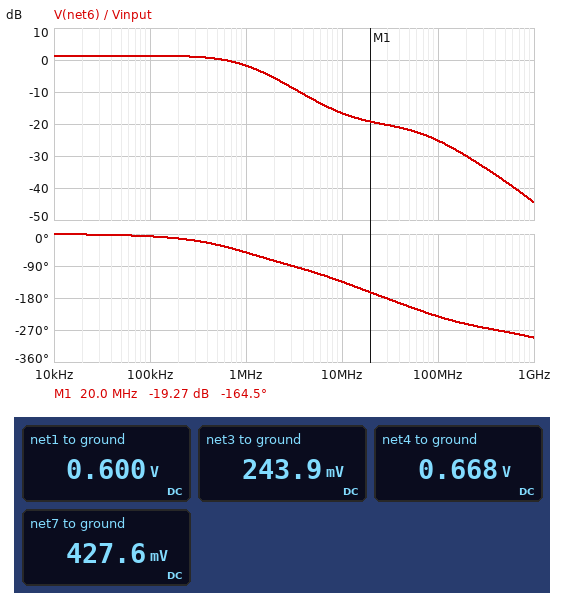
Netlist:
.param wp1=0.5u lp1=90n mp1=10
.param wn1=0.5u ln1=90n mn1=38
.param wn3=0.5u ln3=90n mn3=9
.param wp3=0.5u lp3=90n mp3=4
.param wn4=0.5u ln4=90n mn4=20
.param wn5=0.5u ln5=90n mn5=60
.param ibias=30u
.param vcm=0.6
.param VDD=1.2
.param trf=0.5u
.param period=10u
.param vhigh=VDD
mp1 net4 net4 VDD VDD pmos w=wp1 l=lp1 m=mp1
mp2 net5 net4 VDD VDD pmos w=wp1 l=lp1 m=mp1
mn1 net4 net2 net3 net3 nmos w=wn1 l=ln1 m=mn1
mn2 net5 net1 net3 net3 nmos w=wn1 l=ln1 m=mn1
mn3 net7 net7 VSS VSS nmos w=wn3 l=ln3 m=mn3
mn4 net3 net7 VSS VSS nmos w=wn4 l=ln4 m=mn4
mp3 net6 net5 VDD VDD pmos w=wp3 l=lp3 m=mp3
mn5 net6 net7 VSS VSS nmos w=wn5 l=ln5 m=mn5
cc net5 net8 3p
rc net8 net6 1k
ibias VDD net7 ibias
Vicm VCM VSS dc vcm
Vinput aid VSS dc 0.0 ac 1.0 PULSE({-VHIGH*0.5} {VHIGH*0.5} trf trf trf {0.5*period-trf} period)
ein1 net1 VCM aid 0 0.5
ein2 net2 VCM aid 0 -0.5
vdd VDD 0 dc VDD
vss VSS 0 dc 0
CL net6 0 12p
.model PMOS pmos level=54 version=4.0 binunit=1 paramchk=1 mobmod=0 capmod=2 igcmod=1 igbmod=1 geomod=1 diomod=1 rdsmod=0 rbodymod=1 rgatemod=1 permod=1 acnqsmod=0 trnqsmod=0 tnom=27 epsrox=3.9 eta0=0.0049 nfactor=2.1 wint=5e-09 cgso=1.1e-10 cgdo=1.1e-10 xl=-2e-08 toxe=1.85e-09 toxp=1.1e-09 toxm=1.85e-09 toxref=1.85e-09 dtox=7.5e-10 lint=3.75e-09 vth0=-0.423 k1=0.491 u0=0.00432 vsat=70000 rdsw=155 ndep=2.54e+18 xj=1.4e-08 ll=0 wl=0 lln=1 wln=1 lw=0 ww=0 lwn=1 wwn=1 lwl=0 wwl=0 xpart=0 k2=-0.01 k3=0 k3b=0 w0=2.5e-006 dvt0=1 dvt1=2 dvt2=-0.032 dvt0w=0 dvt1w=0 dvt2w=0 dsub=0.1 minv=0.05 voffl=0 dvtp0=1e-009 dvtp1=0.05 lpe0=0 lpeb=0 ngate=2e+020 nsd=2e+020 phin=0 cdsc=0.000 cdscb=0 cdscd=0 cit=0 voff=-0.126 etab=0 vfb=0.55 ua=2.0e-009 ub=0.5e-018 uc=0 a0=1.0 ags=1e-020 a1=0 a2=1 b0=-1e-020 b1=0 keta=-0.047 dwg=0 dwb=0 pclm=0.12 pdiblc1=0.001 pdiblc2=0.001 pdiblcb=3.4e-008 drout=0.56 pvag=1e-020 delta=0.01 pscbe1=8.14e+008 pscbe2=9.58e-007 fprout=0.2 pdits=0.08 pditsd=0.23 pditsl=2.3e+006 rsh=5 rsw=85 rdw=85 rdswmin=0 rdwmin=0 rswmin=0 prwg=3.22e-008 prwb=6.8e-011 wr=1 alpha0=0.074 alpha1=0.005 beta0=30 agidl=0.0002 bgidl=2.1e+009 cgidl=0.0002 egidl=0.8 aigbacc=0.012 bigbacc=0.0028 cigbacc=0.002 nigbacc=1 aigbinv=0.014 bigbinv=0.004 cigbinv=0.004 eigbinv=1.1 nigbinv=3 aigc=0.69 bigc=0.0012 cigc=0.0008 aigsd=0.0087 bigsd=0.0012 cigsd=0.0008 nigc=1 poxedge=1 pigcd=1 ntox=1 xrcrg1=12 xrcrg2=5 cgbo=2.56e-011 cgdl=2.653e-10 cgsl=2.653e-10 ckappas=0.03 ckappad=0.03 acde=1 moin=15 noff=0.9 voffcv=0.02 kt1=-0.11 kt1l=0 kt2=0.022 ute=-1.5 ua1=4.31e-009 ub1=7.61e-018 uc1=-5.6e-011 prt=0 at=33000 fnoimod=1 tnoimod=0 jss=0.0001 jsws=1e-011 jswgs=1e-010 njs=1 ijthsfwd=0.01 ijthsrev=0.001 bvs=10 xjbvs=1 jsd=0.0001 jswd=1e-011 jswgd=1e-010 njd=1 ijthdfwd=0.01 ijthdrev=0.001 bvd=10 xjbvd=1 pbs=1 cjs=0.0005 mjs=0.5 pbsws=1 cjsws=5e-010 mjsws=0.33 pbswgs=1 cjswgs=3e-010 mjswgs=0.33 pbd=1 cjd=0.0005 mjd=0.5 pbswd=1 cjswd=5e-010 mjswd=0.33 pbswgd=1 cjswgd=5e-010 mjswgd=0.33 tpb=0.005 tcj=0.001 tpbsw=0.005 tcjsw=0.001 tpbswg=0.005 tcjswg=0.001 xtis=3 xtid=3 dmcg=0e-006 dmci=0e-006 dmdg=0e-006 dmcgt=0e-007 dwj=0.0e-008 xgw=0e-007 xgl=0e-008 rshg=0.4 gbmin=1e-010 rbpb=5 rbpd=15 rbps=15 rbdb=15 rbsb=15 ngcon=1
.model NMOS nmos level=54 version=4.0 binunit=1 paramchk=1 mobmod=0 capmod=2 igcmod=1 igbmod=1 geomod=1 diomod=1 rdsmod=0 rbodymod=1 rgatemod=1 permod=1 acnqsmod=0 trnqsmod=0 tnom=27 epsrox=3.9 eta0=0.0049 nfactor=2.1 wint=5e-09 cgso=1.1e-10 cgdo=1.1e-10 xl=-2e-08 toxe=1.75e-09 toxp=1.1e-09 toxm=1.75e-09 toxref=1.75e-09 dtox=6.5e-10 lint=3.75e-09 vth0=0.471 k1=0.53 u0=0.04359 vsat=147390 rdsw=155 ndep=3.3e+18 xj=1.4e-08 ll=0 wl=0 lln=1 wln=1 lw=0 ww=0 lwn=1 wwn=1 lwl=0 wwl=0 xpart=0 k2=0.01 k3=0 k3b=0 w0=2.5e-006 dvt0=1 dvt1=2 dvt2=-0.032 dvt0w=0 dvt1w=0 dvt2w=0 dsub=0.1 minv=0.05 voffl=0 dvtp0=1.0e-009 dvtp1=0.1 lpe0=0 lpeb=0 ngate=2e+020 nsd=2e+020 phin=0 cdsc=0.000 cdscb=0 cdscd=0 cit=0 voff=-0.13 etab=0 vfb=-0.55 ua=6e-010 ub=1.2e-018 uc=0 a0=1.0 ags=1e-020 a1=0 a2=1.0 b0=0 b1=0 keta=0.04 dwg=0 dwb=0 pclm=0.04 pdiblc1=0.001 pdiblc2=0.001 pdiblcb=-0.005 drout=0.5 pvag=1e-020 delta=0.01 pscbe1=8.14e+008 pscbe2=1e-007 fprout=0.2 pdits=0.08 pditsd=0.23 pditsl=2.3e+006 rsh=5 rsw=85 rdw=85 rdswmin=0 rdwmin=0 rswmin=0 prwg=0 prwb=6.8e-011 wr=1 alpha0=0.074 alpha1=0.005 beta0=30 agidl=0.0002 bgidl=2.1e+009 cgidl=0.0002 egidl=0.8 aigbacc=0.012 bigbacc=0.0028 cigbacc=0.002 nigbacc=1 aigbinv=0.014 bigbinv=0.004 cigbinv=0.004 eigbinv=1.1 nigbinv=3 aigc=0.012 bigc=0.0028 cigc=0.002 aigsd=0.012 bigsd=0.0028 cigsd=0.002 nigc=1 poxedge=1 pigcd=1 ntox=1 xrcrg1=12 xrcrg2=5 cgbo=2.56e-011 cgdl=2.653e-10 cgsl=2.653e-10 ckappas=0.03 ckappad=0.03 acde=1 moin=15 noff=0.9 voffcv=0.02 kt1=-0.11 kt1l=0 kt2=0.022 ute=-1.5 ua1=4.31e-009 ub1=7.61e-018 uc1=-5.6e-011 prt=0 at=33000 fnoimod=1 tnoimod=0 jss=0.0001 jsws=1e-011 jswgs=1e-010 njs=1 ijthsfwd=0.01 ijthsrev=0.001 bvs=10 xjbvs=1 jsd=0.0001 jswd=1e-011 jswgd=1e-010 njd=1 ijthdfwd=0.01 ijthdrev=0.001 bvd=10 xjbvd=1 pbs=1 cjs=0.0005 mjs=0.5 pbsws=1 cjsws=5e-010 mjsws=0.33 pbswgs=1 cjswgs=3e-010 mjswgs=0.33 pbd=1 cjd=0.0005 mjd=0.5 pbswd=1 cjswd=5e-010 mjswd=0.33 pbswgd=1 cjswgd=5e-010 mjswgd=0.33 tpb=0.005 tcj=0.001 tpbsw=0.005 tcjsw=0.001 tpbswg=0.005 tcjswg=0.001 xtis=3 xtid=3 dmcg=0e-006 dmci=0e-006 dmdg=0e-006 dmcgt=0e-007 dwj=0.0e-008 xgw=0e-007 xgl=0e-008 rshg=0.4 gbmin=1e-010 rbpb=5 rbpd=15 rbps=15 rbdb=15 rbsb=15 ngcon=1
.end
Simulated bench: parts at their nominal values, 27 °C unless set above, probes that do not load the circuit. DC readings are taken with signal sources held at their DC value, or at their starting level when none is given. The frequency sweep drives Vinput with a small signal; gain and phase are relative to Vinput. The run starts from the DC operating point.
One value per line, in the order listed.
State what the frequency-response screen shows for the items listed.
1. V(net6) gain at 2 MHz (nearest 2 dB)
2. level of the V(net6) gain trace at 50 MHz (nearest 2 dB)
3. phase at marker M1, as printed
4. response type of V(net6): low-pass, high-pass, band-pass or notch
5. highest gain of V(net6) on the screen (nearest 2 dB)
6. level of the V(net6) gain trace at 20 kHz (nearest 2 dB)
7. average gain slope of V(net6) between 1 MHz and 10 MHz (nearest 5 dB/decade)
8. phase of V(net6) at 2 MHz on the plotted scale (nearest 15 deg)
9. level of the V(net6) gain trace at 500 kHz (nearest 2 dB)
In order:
-6 dB
-22 dB
-164.5 deg
low-pass
2 dB
2 dB
-15 dB/decade
-75 deg
0 dB
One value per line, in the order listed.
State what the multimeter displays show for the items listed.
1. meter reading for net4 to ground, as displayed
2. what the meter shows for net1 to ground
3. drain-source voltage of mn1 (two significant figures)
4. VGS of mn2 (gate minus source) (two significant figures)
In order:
0.668 V
0.600 V
420 mV
360 mV
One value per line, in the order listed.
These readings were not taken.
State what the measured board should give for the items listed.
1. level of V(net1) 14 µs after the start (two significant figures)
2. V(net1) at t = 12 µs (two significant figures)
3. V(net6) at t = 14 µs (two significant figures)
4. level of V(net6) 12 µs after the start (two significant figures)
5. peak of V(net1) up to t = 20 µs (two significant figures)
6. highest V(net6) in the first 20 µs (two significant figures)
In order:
900 mV
900 mV
810 mV
810 mV
900 mV
810 mV
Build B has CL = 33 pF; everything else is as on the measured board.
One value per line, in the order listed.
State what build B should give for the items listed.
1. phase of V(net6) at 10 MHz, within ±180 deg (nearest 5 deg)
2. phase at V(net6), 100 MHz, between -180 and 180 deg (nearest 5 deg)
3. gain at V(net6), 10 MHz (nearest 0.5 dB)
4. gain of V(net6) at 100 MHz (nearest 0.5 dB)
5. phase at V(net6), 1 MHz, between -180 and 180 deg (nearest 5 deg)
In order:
-150 deg
110 deg
-17.0 dB
-32.5 dB
-55 deg
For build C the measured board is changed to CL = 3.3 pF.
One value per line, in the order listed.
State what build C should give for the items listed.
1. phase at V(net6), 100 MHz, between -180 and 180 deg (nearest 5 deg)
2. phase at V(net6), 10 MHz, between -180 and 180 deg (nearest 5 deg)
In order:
160 deg
-130 deg
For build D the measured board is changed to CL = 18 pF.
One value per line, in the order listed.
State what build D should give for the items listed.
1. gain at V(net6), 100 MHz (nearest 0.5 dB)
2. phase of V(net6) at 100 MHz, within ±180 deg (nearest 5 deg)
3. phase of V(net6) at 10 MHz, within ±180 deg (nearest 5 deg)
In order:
-28.0 dB
120 deg
-140 deg
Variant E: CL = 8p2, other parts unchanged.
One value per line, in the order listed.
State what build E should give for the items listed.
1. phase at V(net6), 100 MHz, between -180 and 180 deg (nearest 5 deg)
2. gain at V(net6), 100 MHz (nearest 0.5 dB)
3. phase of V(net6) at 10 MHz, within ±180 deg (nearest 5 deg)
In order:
140 deg
-23.0 dB
-130 deg
